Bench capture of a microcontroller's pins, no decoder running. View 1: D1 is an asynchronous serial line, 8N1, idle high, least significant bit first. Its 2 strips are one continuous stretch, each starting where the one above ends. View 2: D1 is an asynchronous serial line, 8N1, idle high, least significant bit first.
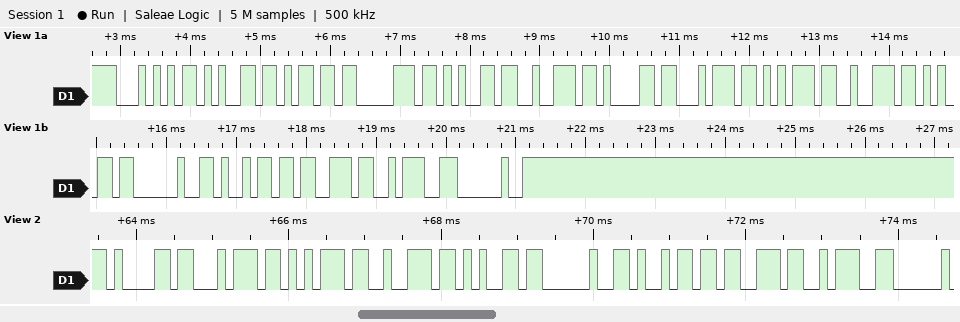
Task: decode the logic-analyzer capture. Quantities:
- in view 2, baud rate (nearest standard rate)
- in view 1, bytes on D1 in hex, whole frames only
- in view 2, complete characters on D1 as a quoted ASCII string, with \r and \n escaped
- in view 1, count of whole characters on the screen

9600 baud
54 65 6D 70 65 72 61 74 75 72 65 20 69 73 3A 20
"ature is:"
16
